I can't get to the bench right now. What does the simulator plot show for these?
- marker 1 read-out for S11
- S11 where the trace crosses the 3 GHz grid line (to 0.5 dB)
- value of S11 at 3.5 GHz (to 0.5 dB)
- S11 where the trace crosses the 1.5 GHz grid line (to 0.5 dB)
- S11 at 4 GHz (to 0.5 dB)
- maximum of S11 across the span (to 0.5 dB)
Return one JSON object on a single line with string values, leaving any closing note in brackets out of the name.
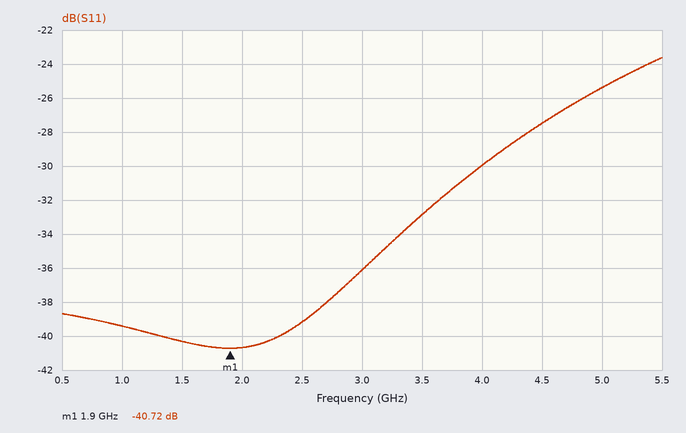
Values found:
{"marker 1 read-out for S11": "-40.72 dB", "S11 where the trace crosses the 3 GHz grid line": "-36.0 dB", "value of S11 at 3.5 GHz": "-33.0 dB", "S11 where the trace crosses the 1.5 GHz grid line": "-40.5 dB", "S11 at 4 GHz": "-30.0 dB", "maximum of S11 across the span": "-23.5 dB"}
